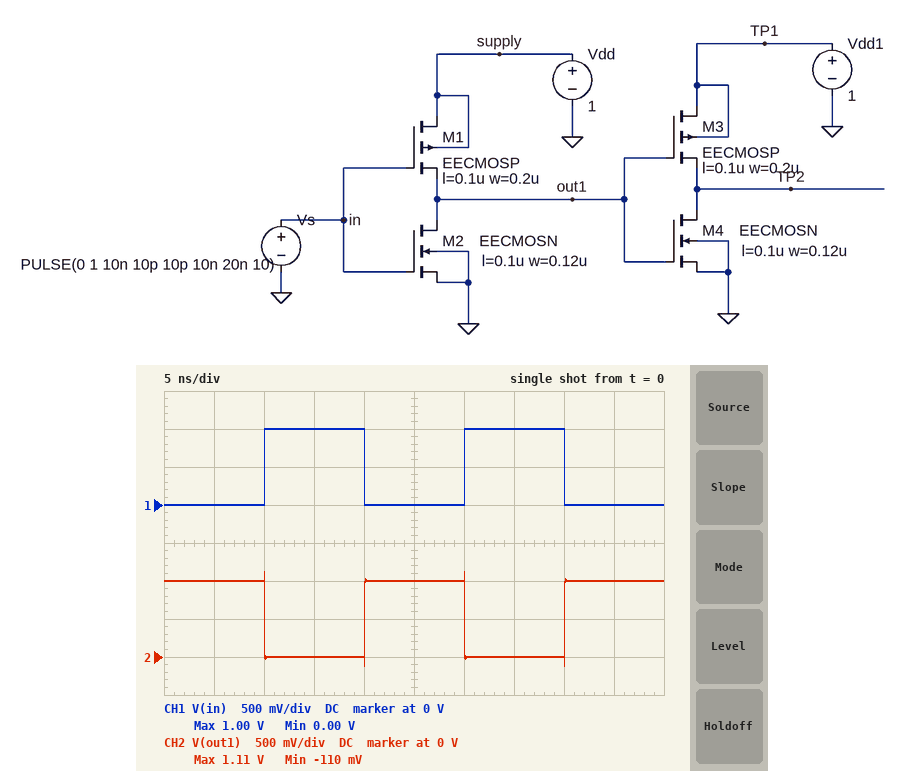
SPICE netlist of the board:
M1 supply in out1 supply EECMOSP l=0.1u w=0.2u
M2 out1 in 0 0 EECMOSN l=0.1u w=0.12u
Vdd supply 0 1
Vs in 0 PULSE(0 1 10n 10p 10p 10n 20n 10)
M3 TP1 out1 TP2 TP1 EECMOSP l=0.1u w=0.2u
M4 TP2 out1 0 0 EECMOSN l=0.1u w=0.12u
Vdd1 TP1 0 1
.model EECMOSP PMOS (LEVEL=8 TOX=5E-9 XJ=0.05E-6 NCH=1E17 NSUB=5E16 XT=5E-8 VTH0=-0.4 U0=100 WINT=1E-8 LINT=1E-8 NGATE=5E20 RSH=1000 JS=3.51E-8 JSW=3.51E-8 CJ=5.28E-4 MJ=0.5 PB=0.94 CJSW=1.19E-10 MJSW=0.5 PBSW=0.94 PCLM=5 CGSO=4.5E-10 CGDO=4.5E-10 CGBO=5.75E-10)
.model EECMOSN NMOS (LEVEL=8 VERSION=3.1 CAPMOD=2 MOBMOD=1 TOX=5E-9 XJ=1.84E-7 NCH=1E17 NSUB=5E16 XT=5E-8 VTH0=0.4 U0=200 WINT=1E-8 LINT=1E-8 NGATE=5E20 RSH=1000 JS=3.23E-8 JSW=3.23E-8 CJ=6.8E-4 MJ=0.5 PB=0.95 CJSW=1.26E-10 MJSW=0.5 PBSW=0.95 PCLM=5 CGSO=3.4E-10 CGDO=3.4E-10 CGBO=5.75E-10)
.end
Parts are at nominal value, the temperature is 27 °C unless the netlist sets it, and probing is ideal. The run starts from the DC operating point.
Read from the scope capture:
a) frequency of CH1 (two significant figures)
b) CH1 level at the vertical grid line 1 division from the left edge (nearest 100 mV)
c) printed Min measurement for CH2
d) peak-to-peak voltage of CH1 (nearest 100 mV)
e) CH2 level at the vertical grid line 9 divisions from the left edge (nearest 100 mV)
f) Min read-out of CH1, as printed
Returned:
50 MHz
0 V
-110 mV
1.0 V
1.0 V
0.00 V
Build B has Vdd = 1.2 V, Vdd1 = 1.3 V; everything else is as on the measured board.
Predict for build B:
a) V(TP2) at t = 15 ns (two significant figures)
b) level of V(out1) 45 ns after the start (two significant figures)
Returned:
1.3 V
1.2 V
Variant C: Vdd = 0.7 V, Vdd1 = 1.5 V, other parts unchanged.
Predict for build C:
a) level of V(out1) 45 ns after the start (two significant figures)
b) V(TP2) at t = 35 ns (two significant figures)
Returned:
700 mV
1.5 V
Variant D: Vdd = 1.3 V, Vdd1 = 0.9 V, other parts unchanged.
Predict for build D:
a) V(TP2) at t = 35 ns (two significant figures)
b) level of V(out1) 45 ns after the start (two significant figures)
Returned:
900 mV
1.3 V
